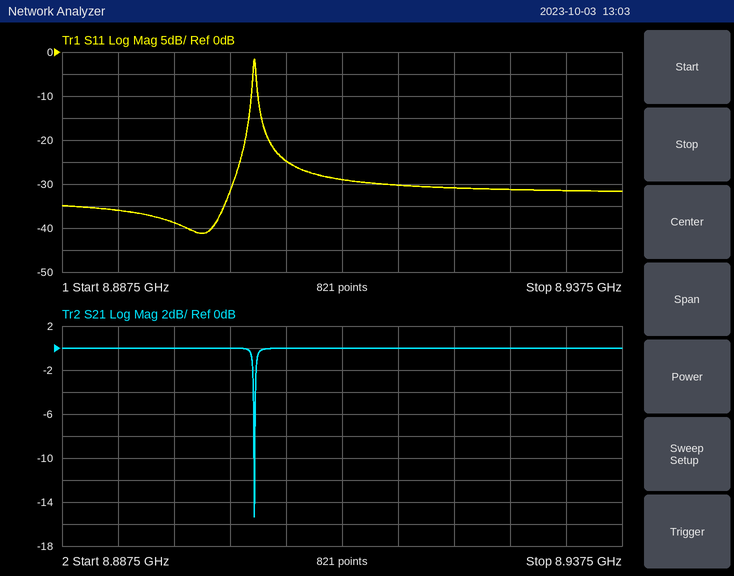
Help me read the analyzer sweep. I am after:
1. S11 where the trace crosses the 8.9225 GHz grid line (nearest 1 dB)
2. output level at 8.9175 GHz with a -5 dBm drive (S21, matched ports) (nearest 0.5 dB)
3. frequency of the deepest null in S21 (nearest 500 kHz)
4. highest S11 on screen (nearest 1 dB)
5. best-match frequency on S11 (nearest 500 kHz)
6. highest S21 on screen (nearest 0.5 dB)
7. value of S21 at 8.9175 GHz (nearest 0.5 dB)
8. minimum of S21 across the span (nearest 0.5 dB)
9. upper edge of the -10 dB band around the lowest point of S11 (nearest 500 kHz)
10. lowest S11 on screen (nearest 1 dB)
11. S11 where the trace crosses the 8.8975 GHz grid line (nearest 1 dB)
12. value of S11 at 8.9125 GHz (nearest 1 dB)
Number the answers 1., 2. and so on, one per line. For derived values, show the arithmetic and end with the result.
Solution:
1. -31 dB
2. -5 dBm + (0.0 dB) = -5.0 dBm
3. 8.9045 GHz
4. -2 dB
5. 8.9000 GHz
6. 0.0 dB
7. 0.0 dB
8. -15.5 dB
9. 8.9045 GHz
10. -41 dB
11. -39 dB
12. -29 dB
